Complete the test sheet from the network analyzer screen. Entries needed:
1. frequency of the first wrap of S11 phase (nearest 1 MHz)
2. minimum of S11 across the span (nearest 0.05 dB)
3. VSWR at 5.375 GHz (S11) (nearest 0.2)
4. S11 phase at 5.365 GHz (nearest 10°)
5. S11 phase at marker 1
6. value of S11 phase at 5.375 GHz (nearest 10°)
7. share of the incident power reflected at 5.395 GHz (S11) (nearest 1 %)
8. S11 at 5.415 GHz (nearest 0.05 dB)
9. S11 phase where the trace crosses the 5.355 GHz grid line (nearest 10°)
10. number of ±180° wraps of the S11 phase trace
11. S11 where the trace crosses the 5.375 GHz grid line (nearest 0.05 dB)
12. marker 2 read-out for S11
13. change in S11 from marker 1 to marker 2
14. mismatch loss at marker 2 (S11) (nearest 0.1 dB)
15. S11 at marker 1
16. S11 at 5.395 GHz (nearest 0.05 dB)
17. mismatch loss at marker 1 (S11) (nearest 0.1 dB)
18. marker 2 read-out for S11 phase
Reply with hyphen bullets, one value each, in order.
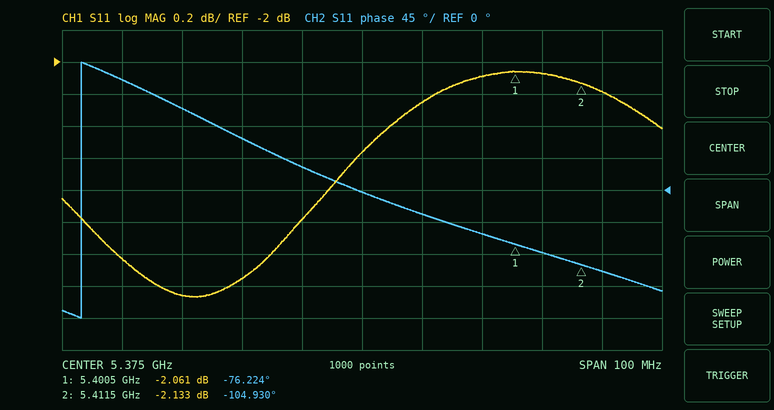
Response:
- 5.328 GHz
- -3.45 dB
- 6.8
- 30°
- -76.224°
- 0°
- 62 %
- -2.20 dB
- 70°
- 1
- -2.55 dB
- -2.133 dB
- -0.072 dB
- 4.1 dB
- -2.061 dB
- -2.10 dB
- 4.2 dB
- -104.930°
